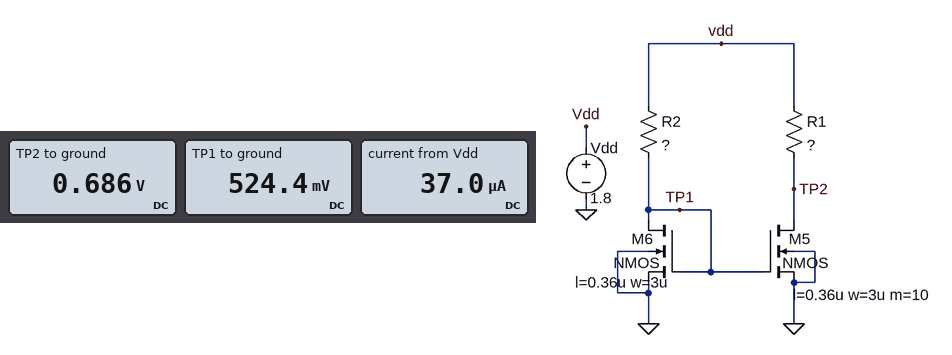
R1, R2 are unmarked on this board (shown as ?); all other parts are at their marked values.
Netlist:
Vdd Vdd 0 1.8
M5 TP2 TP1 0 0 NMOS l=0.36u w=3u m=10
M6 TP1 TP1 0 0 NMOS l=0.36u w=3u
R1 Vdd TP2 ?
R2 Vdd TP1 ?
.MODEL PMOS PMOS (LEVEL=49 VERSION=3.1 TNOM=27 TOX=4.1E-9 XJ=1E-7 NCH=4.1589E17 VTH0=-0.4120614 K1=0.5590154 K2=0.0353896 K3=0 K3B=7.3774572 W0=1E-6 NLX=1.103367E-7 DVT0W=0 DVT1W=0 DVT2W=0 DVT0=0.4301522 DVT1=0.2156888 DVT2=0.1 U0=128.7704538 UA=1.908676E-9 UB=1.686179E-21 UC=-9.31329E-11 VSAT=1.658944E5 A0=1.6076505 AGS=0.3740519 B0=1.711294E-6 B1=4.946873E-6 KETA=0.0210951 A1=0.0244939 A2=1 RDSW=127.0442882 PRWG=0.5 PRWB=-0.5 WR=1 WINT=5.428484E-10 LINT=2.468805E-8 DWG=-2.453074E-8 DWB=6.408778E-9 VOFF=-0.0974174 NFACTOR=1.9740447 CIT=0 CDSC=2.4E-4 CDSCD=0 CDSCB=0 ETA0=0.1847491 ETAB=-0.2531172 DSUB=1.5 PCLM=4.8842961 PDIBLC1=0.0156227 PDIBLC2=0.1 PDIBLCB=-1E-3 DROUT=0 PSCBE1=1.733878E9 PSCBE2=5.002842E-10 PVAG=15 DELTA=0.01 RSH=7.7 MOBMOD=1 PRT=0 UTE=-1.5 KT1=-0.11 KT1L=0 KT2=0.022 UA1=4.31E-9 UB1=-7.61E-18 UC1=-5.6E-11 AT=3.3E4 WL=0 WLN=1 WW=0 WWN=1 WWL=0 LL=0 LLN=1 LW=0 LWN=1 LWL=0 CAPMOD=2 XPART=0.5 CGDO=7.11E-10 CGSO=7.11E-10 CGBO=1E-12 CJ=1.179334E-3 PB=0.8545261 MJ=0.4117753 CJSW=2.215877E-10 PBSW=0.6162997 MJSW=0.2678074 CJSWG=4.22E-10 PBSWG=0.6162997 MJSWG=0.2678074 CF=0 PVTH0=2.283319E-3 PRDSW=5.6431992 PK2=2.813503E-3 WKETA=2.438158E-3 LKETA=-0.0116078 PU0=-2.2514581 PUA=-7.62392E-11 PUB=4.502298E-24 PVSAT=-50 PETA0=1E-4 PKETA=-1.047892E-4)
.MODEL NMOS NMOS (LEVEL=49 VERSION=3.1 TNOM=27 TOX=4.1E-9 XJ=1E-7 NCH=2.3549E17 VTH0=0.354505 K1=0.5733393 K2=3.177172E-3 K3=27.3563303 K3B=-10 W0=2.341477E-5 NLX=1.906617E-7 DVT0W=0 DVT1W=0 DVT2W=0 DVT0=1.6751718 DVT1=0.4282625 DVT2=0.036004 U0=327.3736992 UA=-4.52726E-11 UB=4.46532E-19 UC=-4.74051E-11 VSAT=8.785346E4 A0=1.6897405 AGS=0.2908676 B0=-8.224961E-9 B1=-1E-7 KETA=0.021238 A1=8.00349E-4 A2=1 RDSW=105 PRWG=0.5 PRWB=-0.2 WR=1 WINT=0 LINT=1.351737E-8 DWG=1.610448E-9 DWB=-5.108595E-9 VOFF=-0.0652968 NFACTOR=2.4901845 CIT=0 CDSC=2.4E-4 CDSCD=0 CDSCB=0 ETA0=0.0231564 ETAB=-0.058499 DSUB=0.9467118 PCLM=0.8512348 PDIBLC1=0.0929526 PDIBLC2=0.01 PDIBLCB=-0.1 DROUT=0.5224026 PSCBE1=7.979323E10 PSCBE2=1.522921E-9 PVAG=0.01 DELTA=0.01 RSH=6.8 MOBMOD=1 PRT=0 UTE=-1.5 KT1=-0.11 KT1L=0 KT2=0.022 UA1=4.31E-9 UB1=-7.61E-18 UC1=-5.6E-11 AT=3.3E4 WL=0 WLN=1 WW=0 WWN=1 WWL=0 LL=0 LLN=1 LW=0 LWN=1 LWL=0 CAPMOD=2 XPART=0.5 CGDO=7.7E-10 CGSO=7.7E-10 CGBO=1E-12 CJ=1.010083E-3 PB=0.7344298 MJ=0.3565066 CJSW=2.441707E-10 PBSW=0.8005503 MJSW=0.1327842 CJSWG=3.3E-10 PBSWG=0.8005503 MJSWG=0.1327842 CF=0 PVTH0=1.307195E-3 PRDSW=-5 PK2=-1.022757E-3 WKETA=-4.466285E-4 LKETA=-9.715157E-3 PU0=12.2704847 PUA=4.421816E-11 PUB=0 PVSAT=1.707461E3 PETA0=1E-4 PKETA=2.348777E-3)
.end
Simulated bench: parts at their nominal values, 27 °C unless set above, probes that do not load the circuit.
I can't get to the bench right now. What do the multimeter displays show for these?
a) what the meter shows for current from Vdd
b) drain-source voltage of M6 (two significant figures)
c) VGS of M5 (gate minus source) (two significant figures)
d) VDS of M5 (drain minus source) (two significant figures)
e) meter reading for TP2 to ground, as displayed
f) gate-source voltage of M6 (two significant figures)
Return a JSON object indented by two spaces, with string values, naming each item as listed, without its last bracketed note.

{
  "what the meter shows for current from Vdd": "37.0 µA",
  "drain-source voltage of M6": "520 mV",
  "VGS of M5 (gate minus source)": "520 mV",
  "VDS of M5 (drain minus source)": "690 mV",
  "meter reading for TP2 to ground, as displayed": "0.686 V",
  "gate-source voltage of M6": "520 mV"
}
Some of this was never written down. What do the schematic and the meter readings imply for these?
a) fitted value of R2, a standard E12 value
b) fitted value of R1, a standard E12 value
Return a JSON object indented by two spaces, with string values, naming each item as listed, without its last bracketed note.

{
  "fitted value of R2, a standard E12 value": "390 kΩ",
  "fitted value of R1, a standard E12 value": "33 kΩ"
}
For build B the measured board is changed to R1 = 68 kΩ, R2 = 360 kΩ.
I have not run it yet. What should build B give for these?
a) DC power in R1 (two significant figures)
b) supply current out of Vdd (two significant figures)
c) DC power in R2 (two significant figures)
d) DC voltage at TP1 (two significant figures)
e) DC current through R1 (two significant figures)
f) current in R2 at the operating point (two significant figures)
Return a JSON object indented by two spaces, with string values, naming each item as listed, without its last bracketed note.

{
  "DC power in R1": "45 µW",
  "supply current out of Vdd": "29 µA",
  "DC power in R2": "4.5 µW",
  "DC voltage at TP1": "530 mV",
  "DC current through R1": "26 µA",
  "current in R2 at the operating point": "3.5 µA"
}
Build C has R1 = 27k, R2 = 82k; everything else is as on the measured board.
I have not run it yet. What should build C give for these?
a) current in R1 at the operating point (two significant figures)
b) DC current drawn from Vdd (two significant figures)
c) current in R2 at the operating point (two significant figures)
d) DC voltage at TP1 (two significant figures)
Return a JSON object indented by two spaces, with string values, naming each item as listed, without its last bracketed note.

{
  "current in R1 at the operating point": "65 µA",
  "DC current drawn from Vdd": "80 µA",
  "current in R2 at the operating point": "15 µA",
  "DC voltage at TP1": "600 mV"
}
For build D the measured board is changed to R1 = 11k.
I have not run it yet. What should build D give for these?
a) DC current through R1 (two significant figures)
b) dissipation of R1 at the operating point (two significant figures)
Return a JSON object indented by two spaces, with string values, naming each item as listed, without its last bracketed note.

{
  "DC current through R1": "38 µA",
  "dissipation of R1 at the operating point": "16 µW"
}
